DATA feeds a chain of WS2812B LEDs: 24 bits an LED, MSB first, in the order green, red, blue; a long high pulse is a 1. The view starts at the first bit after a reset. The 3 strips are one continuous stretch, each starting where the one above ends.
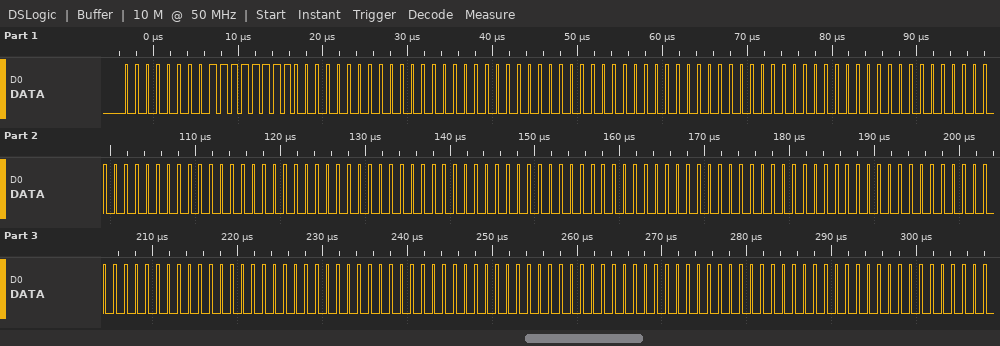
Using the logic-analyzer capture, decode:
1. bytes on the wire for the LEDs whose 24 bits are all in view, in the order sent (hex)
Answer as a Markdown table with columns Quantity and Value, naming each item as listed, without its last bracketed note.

| Quantity | Value |
|---|---|
| bytes on the wire for the LEDs whose 24 bits are all in view, in the order sent | 00 FF 00 00 00 00 00 00 00 00 00 00 00 00 00 00 00 00 00 00 00 00 00 00 00 00 00 00 00 00 |
